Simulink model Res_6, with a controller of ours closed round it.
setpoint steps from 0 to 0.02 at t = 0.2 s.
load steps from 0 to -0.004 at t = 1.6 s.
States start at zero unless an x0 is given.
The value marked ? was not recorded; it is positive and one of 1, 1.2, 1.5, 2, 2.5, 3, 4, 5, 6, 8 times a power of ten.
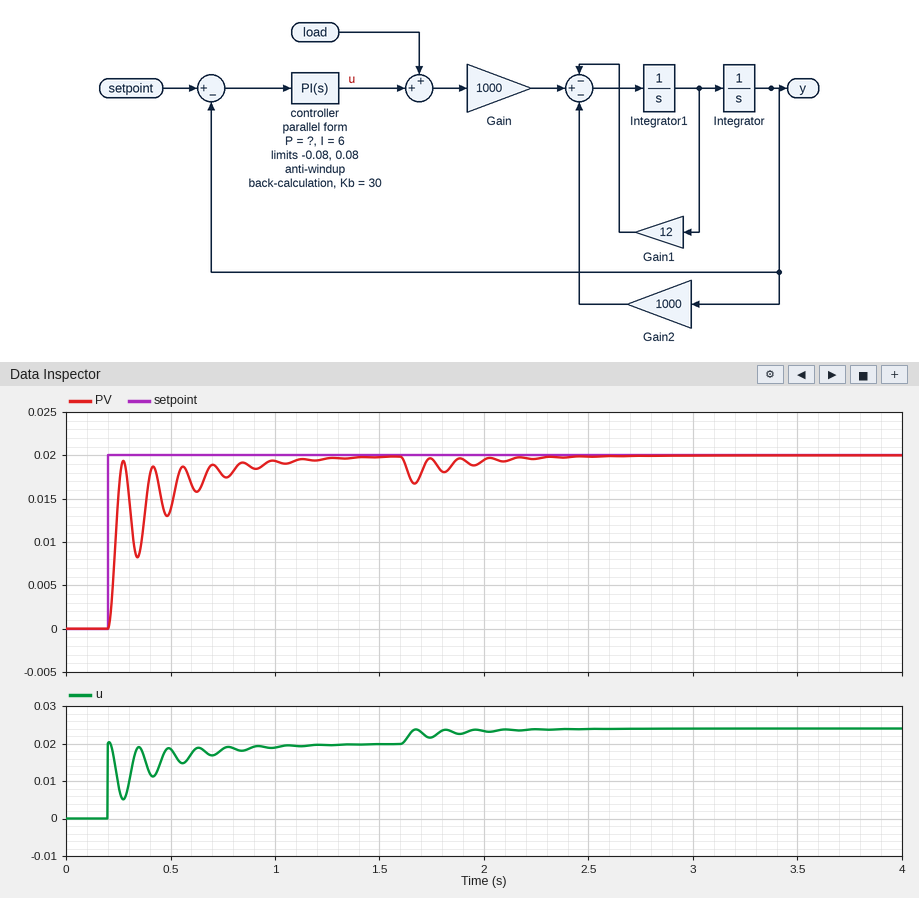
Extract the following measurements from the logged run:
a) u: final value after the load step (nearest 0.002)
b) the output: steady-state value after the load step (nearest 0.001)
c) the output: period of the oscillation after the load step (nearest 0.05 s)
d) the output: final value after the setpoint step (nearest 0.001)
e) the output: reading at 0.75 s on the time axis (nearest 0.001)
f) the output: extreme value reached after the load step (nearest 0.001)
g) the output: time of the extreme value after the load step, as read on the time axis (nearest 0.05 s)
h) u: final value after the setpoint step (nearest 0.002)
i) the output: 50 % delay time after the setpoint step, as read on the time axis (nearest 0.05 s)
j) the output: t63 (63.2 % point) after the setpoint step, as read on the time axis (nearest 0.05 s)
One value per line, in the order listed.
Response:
0.024
0.020
0.15 s
0.020
0.018
0.017
1.65 s
0.020
0.25 s
0.25 s
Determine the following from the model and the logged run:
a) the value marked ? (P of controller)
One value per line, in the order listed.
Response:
1
